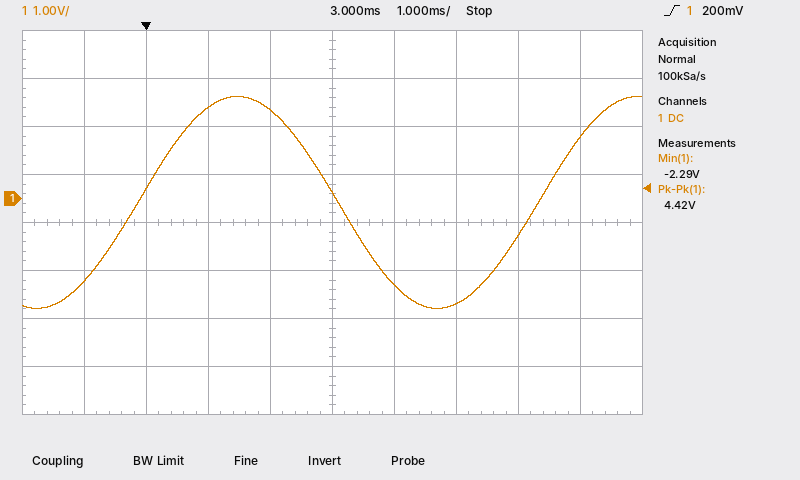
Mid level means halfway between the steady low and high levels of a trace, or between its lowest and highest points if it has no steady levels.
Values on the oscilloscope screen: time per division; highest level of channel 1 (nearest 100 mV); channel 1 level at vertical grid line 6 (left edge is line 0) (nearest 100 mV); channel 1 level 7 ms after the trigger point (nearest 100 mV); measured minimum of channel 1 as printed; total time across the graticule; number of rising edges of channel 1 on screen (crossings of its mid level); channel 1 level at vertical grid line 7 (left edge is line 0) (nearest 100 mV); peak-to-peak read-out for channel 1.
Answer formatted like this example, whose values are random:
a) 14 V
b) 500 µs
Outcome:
a) 1 ms
b) 2.1 V
c) -1.8 V
d) 1.3 V
e) -2.29 V
f) 10 ms
g) 2
h) -2.2 V
i) 4.42 V
